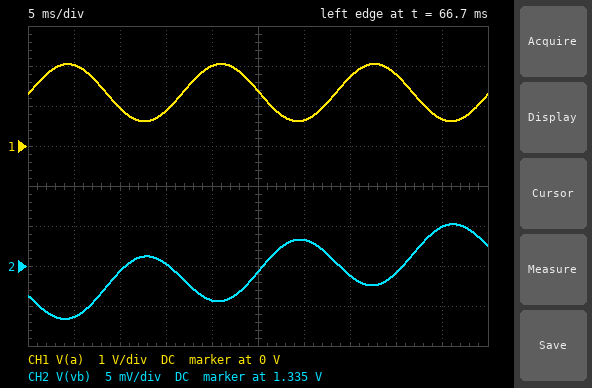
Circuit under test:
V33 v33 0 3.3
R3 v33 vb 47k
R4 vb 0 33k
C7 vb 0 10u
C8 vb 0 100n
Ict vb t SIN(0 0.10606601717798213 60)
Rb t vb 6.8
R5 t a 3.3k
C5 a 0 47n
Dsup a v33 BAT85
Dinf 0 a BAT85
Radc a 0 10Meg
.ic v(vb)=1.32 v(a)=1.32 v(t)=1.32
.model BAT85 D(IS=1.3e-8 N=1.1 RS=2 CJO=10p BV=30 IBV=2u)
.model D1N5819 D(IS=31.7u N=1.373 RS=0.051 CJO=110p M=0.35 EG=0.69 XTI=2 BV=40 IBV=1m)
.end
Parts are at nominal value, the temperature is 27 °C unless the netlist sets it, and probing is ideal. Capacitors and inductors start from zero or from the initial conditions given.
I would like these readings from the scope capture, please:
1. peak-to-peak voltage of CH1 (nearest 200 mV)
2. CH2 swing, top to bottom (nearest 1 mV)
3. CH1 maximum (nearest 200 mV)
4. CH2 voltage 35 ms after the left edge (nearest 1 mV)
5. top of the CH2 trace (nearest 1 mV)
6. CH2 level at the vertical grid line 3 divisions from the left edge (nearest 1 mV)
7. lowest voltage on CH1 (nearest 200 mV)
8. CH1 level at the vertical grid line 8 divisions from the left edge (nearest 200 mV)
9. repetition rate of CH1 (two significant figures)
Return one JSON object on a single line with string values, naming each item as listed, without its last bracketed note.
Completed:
{"peak-to-peak voltage of CH1": "1.4 V", "CH2 swing, top to bottom": "12 mV", "CH1 maximum": "2.0 V", "CH2 voltage 35 ms after the left edge": "1.334 V", "top of the CH2 trace": "1.340 V", "CH2 level at the vertical grid line 3 divisions from the left edge": "1.335 V", "lowest voltage on CH1": "600 mV", "CH1 level at the vertical grid line 8 divisions from the left edge": "1.8 V", "repetition rate of CH1": "60 Hz"}
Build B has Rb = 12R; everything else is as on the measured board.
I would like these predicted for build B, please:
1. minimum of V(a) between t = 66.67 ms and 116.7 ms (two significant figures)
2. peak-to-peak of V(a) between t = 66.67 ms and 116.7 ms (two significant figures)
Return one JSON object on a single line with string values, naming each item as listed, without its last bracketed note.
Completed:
{"minimum of V(a) between t = 66.67 ms and 116.7 ms": "68 mV", "peak-to-peak of V(a) between t = 66.67 ms and 116.7 ms": "2.5 V"}
